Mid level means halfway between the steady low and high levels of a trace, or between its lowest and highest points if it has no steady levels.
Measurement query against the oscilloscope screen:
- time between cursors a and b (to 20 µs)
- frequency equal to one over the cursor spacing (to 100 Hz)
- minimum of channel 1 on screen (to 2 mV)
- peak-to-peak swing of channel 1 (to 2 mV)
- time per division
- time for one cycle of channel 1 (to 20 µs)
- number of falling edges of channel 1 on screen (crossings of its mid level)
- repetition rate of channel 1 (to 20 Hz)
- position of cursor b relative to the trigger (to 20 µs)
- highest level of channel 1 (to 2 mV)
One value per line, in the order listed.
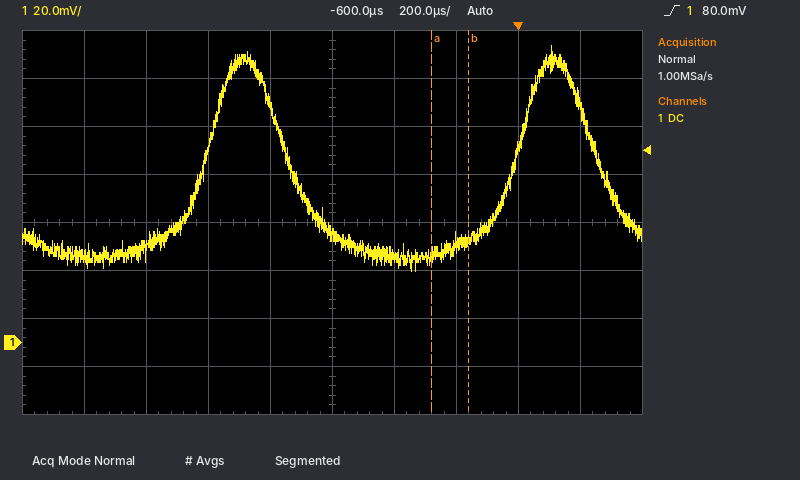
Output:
120 µs
8.3 kHz
30 mV
94 mV
200 µs
1.00 ms
2
1.00 kHz
-160 µs
124 mV
